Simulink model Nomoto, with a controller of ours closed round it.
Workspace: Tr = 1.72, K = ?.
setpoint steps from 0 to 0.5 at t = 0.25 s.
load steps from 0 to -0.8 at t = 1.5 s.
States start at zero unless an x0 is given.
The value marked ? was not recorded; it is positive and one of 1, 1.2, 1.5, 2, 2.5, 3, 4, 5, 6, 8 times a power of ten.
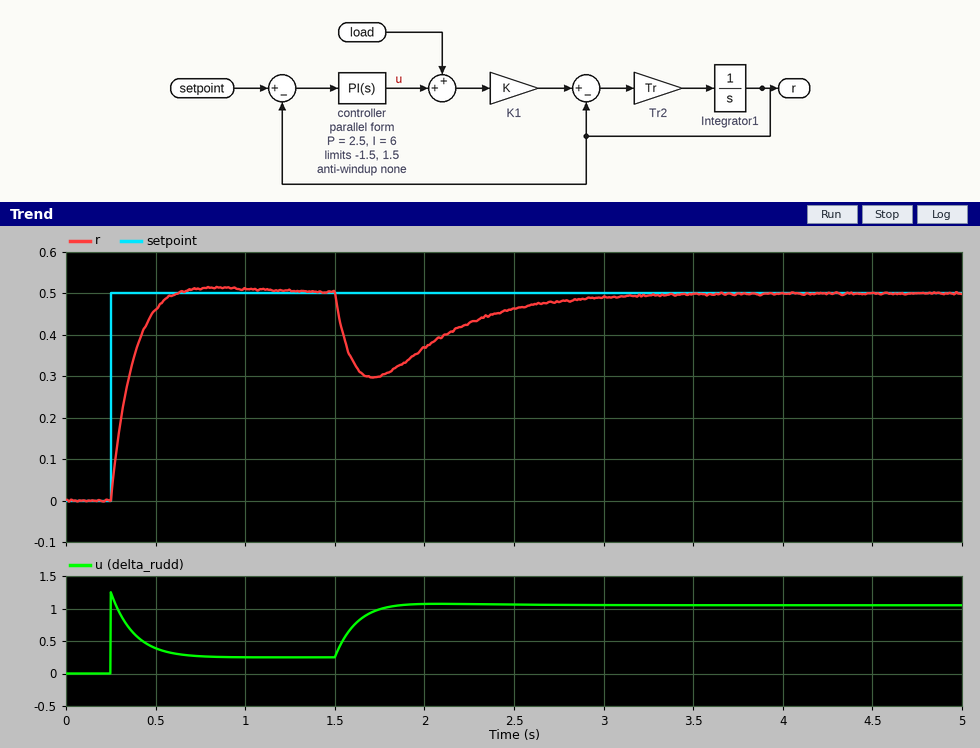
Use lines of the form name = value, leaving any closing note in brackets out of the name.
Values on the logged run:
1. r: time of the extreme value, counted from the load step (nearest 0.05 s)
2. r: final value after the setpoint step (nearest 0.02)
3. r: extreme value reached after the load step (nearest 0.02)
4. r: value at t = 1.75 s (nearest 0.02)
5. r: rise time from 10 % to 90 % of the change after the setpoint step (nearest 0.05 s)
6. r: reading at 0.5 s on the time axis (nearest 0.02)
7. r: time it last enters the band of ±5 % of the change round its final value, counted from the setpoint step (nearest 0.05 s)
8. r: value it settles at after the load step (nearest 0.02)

r: time of the extreme value, counted from the load step = 0.20 s
r: final value after the setpoint step = 0.50
r: extreme value reached after the load step = 0.30
r: value at t = 1.75 s = 0.30
r: rise time from 10 % to 90 % of the change after the setpoint step = 0.20 s
r: reading at 0.5 s on the time axis = 0.46
r: time it last enters the band of ±5 % of the change round its final value, counted from the setpoint step = 0.30 s
r: value it settles at after the load step = 0.50
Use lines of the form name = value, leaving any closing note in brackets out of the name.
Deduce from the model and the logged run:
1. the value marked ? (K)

the value marked ? = 2
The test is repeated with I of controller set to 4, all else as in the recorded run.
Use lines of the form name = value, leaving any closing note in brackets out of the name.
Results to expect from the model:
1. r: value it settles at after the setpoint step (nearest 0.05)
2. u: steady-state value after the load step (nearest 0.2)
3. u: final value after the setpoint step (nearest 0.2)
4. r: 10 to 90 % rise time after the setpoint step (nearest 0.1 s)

r: value it settles at after the setpoint step = 0.50
u: steady-state value after the load step = 1.0
u: final value after the setpoint step = 0.2
r: 10 to 90 % rise time after the setpoint step = 0.3 s
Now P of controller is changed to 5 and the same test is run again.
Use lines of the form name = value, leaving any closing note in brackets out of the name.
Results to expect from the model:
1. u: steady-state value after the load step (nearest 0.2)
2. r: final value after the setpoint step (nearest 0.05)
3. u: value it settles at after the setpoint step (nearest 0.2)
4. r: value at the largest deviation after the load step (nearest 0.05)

u: steady-state value after the load step = 1.0
r: final value after the setpoint step = 0.50
u: value it settles at after the setpoint step = 0.2
r: value at the largest deviation after the load step = 0.35
